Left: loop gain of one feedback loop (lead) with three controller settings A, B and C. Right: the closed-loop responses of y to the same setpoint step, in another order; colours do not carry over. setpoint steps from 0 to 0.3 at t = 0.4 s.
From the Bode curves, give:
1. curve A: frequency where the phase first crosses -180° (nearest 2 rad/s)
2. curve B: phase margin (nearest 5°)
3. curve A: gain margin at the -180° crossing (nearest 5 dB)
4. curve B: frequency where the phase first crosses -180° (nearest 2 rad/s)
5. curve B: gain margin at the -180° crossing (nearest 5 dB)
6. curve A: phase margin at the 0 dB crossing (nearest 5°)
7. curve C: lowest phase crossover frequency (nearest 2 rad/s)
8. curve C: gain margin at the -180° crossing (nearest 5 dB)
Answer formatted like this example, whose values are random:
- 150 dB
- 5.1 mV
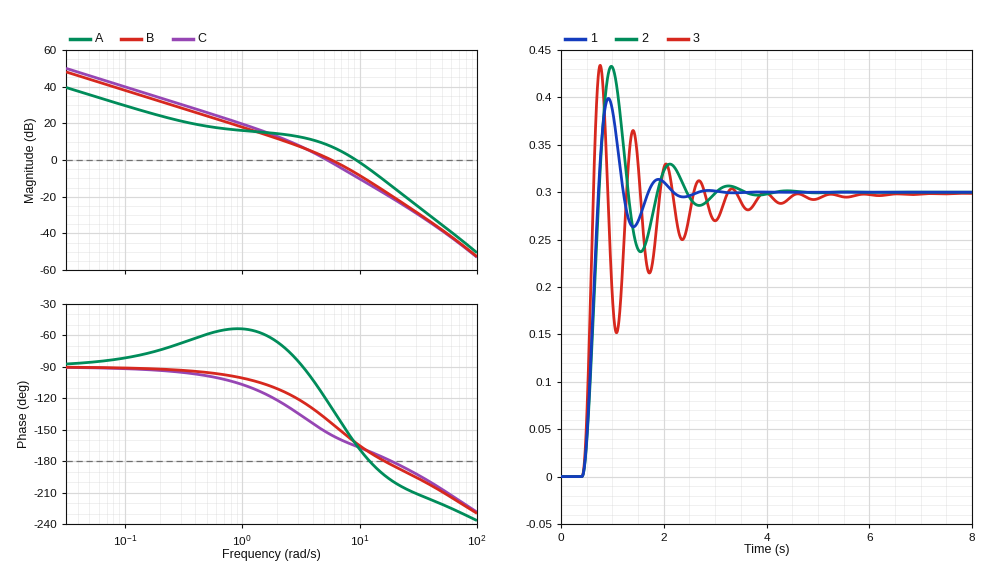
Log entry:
- 12 rad/s
- 35°
- 5 dB
- 16 rad/s
- 15 dB
- 15°
- 18 rad/s
- 20 dB
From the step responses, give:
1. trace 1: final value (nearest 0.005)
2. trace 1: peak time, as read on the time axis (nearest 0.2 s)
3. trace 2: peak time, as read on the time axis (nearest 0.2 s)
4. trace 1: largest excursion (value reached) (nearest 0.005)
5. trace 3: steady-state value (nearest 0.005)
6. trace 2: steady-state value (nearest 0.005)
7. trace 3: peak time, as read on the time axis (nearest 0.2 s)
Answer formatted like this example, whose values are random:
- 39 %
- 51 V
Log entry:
- 0.300
- 1.0 s
- 1.0 s
- 0.400
- 0.300
- 0.300
- 0.8 s
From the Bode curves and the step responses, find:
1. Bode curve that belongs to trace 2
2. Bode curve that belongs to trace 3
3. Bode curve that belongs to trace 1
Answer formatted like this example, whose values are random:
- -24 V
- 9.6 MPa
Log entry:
- C
- A
- B
